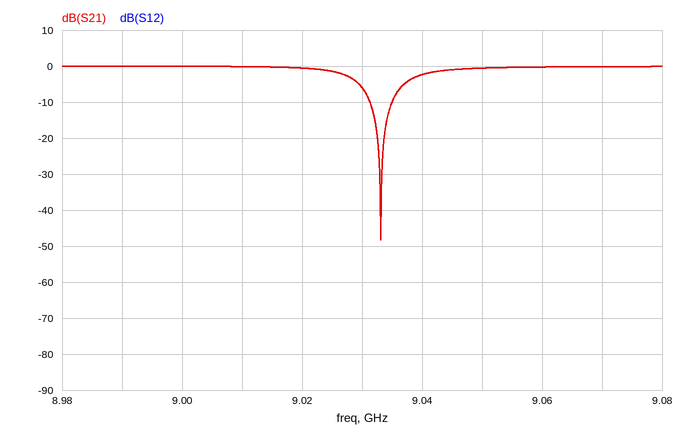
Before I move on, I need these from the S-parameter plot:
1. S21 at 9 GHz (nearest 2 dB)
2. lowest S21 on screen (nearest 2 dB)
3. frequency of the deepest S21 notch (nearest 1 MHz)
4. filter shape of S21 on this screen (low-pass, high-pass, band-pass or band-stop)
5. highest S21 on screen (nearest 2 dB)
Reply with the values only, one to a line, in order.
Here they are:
0 dB
-48 dB
9.033 GHz
band-stop
0 dB
